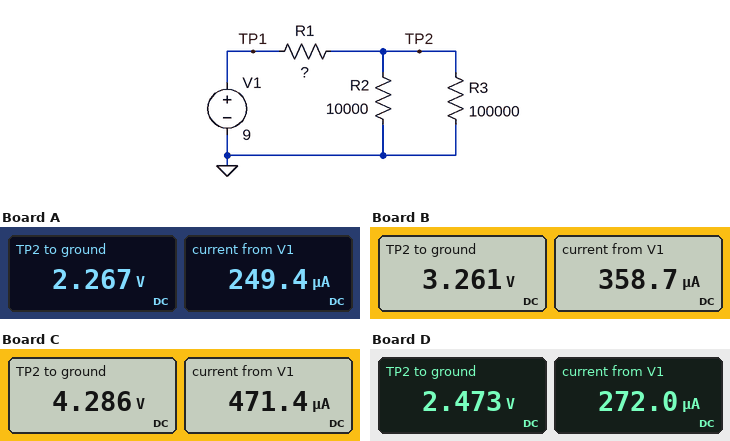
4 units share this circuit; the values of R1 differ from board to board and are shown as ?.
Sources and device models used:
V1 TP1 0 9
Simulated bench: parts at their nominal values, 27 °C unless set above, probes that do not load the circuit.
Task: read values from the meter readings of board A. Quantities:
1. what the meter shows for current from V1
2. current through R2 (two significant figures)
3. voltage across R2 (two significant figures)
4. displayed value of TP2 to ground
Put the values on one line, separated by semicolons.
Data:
249.4 µA; 230 µA; 2.3 V; 2.267 V
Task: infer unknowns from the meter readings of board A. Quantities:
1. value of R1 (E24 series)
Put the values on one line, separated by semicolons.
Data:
27 kΩ
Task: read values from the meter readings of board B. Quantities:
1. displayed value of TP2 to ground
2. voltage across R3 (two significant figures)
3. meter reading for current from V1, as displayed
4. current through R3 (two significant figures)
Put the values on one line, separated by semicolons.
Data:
3.261 V; 3.3 V; 358.7 µA; 33 µA
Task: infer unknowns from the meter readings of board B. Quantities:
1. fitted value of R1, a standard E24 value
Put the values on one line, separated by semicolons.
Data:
16 kΩ
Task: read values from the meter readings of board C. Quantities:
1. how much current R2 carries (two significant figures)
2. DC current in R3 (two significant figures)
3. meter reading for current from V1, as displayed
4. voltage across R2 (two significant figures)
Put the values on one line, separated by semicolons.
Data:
430 µA; 43 µA; 471.4 µA; 4.3 V
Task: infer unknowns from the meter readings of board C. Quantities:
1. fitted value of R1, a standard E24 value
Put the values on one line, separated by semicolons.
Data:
10 kΩ
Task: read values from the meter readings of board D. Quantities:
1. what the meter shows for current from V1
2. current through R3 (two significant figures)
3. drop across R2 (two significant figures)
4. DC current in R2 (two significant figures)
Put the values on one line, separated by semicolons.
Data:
272.0 µA; 25 µA; 2.5 V; 250 µA
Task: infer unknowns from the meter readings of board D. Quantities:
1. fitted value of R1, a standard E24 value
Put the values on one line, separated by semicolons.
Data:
24 kΩ
